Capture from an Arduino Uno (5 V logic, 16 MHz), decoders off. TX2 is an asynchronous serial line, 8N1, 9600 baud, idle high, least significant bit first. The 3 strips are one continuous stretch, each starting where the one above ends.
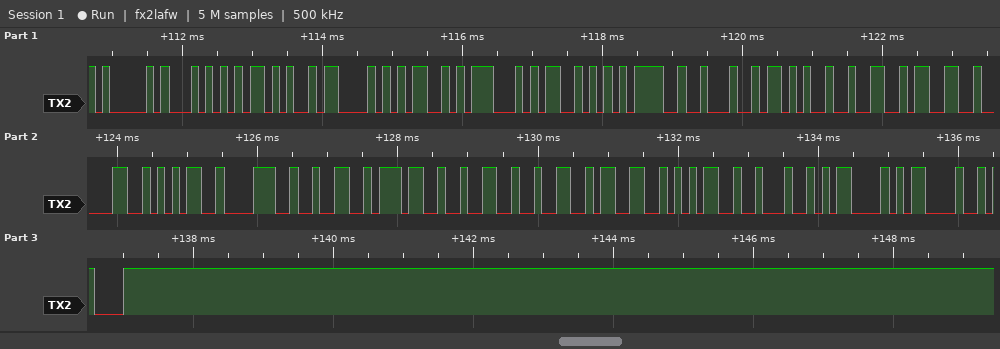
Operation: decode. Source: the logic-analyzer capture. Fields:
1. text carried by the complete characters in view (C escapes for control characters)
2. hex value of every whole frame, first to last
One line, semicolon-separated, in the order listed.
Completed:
"AT+CMGS=\"+23058272235\"\r\r\n"; 41 54 2B 43 4D 47 53 3D 22 2B 32 33 30 35 38 32 37 32 32 33 35 22 0D 0D 0A
